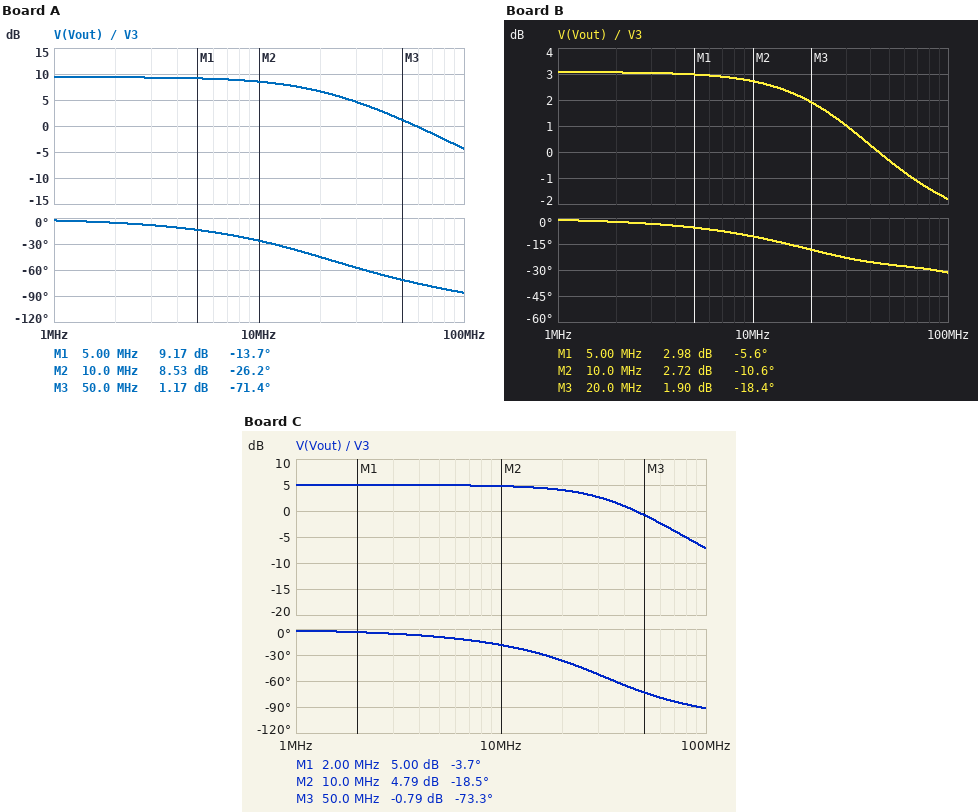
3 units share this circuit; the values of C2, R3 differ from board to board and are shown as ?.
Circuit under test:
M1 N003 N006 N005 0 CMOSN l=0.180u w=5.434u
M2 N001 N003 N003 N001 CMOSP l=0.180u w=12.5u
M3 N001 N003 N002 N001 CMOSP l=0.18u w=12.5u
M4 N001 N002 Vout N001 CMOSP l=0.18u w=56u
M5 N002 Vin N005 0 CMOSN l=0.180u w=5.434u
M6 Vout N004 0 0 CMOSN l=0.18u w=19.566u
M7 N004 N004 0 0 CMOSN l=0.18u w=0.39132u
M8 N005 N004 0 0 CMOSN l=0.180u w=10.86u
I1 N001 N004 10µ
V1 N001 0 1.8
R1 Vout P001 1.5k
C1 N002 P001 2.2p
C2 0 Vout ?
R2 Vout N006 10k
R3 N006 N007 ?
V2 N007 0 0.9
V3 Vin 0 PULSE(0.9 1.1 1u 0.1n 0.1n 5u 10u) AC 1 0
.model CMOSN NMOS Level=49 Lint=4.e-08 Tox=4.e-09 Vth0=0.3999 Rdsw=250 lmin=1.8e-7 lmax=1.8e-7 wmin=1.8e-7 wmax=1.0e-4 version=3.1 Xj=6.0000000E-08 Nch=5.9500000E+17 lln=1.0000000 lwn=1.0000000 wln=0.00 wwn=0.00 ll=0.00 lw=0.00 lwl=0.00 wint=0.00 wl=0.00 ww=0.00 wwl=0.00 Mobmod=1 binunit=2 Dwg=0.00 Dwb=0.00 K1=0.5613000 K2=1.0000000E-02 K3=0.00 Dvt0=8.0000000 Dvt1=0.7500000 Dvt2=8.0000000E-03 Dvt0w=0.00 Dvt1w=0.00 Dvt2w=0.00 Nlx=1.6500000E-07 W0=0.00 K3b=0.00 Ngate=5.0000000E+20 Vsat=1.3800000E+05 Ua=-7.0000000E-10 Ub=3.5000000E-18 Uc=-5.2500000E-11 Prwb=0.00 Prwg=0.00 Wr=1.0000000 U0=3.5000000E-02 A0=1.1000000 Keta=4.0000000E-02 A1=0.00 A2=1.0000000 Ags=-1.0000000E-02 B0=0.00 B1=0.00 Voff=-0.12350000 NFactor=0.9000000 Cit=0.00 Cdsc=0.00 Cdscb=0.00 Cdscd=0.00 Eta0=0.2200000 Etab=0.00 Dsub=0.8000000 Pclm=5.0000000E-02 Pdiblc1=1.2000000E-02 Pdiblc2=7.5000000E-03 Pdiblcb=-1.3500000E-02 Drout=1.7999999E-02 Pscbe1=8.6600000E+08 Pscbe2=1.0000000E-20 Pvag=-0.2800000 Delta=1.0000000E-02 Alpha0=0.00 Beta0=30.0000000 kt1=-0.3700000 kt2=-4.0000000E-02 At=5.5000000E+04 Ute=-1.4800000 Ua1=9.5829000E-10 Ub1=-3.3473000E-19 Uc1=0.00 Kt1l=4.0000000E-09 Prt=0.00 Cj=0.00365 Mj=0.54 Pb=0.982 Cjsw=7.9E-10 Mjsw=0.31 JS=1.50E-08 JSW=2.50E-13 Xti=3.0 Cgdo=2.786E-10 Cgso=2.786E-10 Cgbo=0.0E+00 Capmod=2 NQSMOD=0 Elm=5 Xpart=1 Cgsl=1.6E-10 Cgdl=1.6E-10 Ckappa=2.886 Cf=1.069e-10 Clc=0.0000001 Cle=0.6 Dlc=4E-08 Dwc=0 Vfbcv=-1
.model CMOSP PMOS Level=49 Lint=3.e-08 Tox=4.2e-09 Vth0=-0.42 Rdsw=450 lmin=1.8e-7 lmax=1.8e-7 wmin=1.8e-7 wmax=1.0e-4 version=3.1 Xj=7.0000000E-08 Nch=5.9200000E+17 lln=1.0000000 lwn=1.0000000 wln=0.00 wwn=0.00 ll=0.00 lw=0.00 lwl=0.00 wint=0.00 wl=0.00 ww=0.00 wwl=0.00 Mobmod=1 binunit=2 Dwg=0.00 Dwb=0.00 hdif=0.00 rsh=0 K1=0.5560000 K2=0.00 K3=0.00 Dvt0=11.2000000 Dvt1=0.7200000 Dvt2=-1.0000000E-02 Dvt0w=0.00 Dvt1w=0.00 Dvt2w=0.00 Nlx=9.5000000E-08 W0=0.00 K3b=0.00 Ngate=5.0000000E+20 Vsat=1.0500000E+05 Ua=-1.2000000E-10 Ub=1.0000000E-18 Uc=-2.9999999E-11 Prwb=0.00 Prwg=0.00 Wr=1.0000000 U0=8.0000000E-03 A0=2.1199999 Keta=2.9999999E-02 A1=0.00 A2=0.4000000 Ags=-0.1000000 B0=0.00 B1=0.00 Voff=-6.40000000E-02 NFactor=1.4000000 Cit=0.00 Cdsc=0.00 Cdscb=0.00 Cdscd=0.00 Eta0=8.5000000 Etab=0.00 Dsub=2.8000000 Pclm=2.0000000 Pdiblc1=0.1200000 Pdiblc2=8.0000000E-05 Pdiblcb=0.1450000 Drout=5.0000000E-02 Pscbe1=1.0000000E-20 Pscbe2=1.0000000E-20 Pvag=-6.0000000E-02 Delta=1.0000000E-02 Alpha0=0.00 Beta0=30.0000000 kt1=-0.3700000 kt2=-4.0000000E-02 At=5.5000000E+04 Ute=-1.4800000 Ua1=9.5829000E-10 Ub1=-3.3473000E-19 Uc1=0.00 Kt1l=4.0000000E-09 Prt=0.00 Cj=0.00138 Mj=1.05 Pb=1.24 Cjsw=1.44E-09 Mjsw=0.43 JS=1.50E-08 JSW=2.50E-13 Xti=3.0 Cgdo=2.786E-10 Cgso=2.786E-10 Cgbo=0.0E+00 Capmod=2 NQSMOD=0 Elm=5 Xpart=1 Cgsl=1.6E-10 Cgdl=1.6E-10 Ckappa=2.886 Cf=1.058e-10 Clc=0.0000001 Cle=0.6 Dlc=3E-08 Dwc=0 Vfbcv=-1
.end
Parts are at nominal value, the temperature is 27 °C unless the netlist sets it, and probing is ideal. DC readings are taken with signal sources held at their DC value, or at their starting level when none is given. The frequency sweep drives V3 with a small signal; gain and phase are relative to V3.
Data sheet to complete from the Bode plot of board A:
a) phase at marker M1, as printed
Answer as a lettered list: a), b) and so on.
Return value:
a) -13.7 deg
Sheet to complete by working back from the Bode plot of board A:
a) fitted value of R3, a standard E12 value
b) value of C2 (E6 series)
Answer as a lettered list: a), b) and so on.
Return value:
a) 4.7 kΩ
b) 22 pF
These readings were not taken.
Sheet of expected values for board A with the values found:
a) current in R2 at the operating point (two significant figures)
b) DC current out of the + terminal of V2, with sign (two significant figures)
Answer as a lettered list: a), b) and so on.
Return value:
a) 160 nA
b) -160 nA
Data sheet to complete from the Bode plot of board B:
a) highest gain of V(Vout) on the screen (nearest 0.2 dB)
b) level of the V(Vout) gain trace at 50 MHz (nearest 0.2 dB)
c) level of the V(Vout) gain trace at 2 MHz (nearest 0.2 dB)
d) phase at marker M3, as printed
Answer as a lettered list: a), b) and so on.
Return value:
a) 3.0 dB
b) -0.4 dB
c) 3.0 dB
d) -18.4 deg
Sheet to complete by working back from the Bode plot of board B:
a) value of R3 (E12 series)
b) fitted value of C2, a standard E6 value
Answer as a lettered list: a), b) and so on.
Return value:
a) 22 kΩ
b) 4.7 pF
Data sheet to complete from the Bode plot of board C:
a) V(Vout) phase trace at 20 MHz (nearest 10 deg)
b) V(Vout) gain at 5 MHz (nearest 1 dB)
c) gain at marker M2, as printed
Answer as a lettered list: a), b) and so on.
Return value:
a) -40 deg
b) 5 dB
c) 4.79 dB
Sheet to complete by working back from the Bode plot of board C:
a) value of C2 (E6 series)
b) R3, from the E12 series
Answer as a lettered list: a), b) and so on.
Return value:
a) 33 pF
b) 12 kΩ
